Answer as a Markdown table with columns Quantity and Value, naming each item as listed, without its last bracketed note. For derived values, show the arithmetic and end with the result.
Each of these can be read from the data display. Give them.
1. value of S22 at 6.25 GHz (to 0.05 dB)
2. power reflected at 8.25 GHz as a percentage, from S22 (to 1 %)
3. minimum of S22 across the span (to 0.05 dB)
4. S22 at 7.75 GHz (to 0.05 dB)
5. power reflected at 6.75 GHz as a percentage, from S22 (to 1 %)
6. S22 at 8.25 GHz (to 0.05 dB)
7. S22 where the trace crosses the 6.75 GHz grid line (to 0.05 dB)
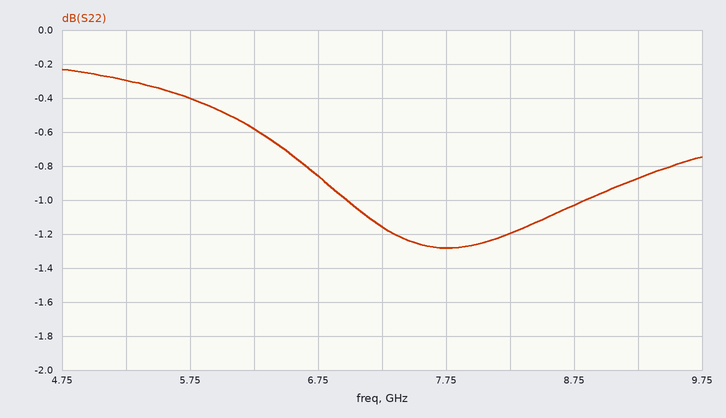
| Quantity | Value |
|---|---|
| value of S22 at 6.25 GHz | -0.60 dB |
| power reflected at 8.25 GHz as a percentage, from S22 | 10^(-1.2/10) ≈ 76 % |
| minimum of S22 across the span | -1.30 dB |
| S22 at 7.75 GHz | -1.30 dB |
| power reflected at 6.75 GHz as a percentage, from S22 | 10^(-0.85/10) ≈ 82 % |
| S22 at 8.25 GHz | -1.20 dB |
| S22 where the trace crosses the 6.75 GHz grid line | -0.85 dB |
